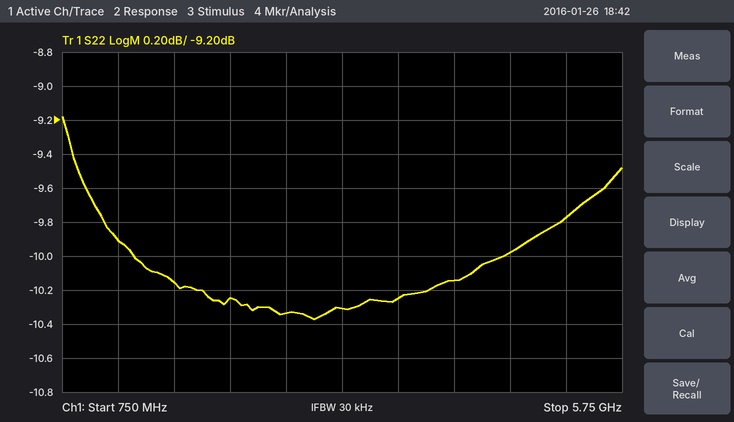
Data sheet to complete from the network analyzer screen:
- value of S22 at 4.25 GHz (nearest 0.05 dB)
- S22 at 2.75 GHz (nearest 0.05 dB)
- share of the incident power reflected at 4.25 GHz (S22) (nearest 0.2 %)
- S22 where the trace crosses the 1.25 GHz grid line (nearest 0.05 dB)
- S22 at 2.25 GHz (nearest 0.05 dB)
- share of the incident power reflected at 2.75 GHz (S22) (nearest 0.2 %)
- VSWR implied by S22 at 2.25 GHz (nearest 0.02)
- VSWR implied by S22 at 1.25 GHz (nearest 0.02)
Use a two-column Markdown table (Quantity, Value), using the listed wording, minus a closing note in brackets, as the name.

| Quantity | Value |
|---|---|
| value of S22 at 4.25 GHz | -10.15 dB |
| S22 at 2.75 GHz | -10.35 dB |
| share of the incident power reflected at 4.25 GHz (S22) | 9.6 % |
| S22 where the trace crosses the 1.25 GHz grid line | -9.90 dB |
| S22 at 2.25 GHz | -10.25 dB |
| share of the incident power reflected at 2.75 GHz (S22) | 9.2 % |
| VSWR implied by S22 at 2.25 GHz | 1.88 |
| VSWR implied by S22 at 1.25 GHz | 1.94 |
